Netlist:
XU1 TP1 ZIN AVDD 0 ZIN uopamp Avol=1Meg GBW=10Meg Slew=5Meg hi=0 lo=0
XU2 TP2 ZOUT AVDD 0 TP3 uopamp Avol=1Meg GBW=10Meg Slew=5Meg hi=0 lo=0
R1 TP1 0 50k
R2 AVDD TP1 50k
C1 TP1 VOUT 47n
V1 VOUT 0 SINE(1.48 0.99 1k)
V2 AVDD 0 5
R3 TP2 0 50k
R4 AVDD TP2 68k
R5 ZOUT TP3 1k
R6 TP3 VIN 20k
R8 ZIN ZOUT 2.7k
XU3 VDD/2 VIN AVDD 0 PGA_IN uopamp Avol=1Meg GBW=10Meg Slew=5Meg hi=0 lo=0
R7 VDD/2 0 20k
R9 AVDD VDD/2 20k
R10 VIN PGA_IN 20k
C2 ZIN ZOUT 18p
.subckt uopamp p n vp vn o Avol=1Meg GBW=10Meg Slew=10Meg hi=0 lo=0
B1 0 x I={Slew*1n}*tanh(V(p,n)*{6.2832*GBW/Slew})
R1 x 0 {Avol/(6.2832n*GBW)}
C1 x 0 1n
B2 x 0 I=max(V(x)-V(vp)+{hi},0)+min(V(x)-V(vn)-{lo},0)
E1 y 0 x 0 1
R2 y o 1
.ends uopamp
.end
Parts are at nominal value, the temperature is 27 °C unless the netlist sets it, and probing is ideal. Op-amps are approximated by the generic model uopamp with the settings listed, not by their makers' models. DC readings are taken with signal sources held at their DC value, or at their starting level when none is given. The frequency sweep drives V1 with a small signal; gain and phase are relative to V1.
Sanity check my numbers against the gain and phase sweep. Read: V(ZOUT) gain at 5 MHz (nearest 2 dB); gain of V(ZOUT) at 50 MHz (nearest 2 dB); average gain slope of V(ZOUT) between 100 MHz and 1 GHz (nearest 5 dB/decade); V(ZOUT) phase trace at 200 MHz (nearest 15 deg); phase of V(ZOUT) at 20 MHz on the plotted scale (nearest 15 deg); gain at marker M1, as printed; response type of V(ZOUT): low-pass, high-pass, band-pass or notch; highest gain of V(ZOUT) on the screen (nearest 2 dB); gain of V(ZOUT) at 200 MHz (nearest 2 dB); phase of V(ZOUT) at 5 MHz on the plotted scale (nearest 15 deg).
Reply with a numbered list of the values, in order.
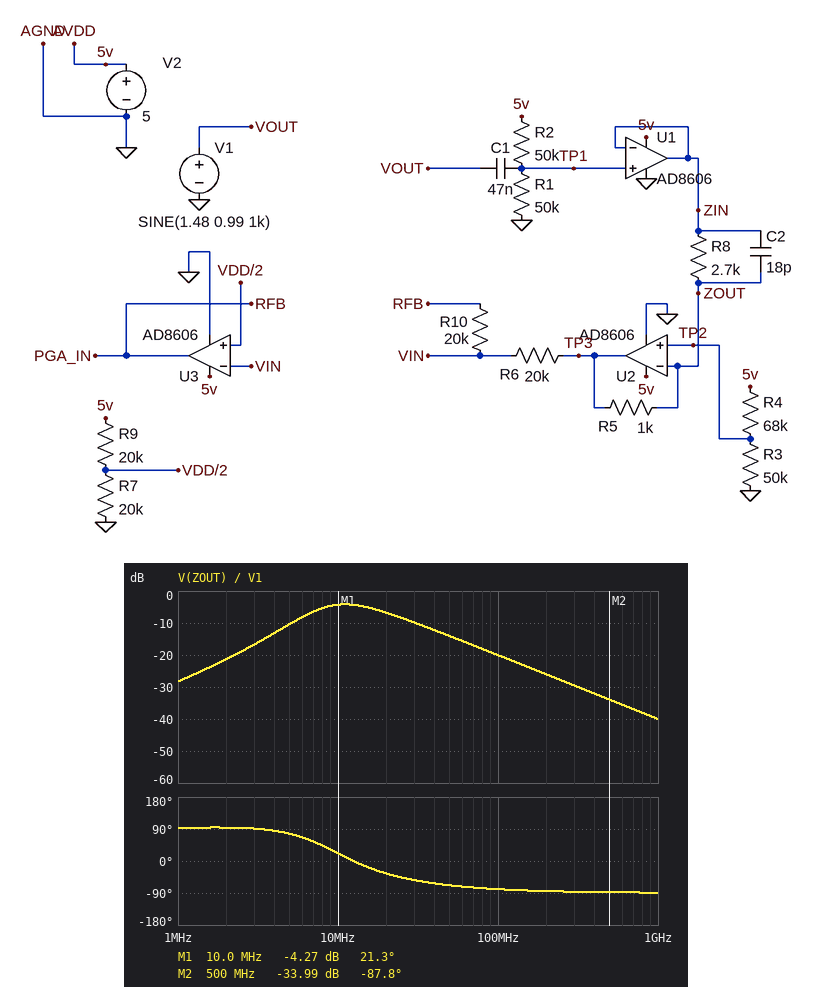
1. -10 dB
2. -14 dB
3. -20 dB/decade
4. -90 deg
5. -30 deg
6. -4.27 dB
7. band-pass
8. -4 dB
9. -26 dB
10. 75 deg
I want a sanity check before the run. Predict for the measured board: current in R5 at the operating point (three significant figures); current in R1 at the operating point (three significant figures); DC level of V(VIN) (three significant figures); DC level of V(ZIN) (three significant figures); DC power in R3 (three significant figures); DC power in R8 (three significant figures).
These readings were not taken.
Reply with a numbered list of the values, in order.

1. 141 µA
2. 50.0 µA
3. 2.50 V
4. 2.50 V
5. 89.8 µW
6. 53.9 µW
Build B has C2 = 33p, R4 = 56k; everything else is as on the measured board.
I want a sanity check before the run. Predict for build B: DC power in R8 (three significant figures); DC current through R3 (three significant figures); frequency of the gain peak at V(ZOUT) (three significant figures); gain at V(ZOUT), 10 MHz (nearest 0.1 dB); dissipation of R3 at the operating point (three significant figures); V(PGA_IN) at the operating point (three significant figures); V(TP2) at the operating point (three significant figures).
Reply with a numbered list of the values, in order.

1. 7.42 µW
2. 47.2 µA
3. 7.95 MHz
4. -1.4 dB
5. 111 µW
6. 2.69 V
7. 2.36 V
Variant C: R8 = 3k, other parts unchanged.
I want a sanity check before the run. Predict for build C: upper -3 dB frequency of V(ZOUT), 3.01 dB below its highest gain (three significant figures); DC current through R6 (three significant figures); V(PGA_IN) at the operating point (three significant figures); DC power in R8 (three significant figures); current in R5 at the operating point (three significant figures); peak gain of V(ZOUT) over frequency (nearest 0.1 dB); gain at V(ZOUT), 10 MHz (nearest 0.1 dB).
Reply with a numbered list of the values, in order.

1. 20.9 MHz
2. 25.4 µA
3. 3.01 V
4. 48.5 µW
5. 127 µA
6. -4.0 dB
7. -4.1 dB
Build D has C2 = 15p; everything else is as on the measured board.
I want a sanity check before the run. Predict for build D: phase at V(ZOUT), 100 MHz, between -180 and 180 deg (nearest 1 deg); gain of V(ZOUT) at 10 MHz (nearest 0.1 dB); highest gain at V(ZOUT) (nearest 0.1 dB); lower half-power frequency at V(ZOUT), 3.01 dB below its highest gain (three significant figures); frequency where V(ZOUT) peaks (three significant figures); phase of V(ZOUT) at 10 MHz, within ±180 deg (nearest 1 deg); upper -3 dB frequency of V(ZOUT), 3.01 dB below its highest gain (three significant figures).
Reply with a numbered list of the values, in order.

1. -78 deg
2. -5.6 dB
3. -5.3 dB
4. 6.83 MHz
5. 12.1 MHz
6. 26 deg
7. 23.9 MHz
